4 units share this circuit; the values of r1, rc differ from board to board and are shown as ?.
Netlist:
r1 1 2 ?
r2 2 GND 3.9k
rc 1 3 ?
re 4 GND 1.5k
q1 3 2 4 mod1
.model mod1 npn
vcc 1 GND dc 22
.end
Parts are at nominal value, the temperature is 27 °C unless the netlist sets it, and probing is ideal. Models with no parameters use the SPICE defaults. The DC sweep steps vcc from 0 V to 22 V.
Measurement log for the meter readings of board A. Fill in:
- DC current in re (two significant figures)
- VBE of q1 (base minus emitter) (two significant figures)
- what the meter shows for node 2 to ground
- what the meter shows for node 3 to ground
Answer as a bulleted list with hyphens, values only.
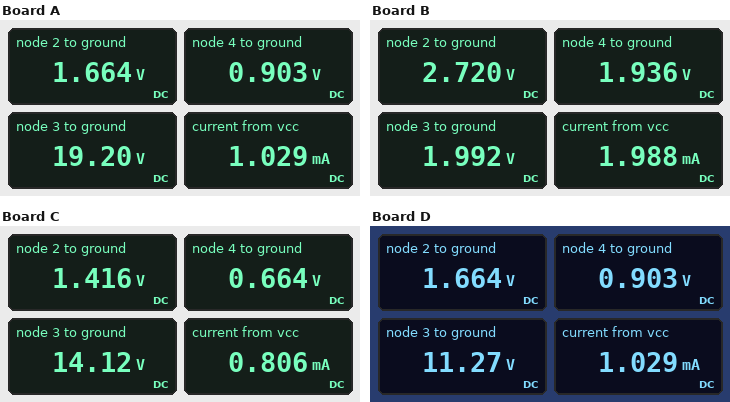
- 600 µA
- 760 mV
- 1.664 V
- 19.20 V
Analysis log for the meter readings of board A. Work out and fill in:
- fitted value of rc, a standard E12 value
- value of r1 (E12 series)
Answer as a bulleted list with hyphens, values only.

- 4.7 kΩ
- 47 kΩ
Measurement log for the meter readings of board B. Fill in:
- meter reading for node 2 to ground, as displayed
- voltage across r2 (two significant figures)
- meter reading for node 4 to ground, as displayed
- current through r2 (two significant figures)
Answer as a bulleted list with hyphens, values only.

- 2.720 V
- 2.7 V
- 1.936 V
- 700 µA
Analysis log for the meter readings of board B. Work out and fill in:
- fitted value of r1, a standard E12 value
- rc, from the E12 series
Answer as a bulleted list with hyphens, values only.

- 22 kΩ
- 18 kΩ
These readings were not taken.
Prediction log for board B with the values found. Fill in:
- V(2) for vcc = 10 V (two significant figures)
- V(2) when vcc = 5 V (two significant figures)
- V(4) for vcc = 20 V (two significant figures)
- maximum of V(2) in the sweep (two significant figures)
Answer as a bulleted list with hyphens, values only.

- 1.5 V
- 750 mV
- 1.7 V
- 2.7 V
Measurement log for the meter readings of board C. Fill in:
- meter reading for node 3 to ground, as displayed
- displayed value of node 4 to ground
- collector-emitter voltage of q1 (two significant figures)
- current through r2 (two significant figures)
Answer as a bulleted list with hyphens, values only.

- 14.12 V
- 0.664 V
- 13 V
- 360 µA
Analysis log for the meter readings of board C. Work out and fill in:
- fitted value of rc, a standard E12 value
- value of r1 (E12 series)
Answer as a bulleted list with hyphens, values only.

- 18 kΩ
- 56 kΩ
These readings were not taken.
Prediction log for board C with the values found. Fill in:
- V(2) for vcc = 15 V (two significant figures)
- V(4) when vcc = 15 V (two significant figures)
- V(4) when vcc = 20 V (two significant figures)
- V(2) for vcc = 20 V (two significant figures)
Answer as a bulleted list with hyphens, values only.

- 970 mV
- 240 mV
- 540 mV
- 1.3 V
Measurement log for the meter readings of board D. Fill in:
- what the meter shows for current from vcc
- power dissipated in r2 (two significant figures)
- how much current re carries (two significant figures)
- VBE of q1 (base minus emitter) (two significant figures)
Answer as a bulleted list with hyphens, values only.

- 1.029 mA
- 710 µW
- 600 µA
- 760 mV
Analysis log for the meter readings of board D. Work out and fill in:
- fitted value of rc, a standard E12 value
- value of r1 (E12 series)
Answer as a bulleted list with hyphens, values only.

- 18 kΩ
- 47 kΩ
